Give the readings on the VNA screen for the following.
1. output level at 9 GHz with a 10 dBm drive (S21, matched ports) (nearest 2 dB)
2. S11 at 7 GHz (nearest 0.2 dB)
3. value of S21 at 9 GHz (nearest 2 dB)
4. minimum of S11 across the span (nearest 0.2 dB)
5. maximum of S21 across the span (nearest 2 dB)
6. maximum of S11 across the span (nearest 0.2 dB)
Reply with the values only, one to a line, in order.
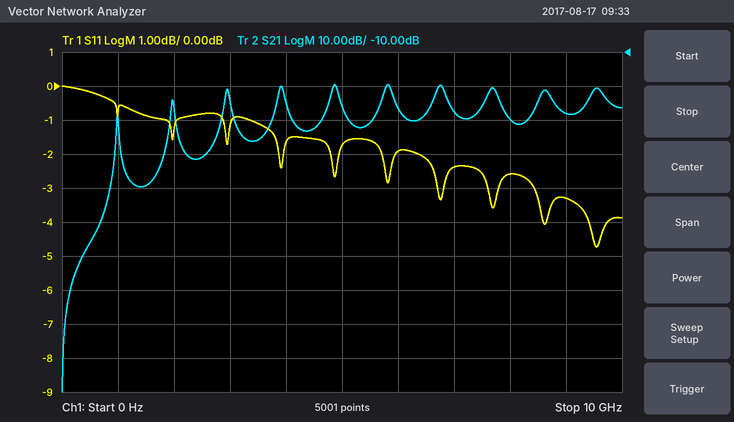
-18 dBm
-2.4 dB
-28 dB
-4.8 dB
-20 dB
0.0 dB
